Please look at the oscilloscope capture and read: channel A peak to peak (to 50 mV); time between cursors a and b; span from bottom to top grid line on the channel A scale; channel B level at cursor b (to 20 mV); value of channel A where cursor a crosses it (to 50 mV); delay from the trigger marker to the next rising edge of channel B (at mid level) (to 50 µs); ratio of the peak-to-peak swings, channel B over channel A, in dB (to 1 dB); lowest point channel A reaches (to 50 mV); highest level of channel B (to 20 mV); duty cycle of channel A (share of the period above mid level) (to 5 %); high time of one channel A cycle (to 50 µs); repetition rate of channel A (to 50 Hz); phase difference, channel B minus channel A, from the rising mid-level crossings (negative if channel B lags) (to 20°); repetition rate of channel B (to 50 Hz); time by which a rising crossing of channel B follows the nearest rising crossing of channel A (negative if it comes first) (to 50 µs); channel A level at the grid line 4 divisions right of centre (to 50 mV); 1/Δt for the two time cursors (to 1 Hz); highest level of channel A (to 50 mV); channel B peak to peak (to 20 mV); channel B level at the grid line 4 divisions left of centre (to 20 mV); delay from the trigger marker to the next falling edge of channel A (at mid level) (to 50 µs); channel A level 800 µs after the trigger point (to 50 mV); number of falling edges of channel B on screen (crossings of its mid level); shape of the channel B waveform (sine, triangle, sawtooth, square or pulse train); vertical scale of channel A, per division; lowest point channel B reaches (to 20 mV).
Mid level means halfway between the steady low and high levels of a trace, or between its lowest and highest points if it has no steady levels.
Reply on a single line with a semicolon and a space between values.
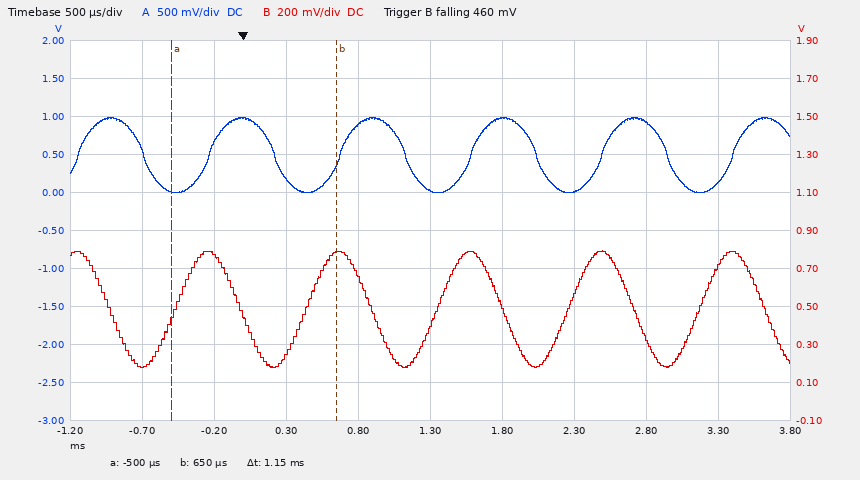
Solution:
1.00 V; 1.15 ms; 5 V; 780 mV; 0 mV; 450 µs; -4 dB; 0 mV; 800 mV; 50 %; 450 µs; 1.10 kHz; +100°; 1.10 kHz; -250 µs; 150 mV; 870 Hz; 1.00 V; 620 mV; 180 mV; 200 µs; 900 mV; 6; sine; 500 mV; 180 mV
